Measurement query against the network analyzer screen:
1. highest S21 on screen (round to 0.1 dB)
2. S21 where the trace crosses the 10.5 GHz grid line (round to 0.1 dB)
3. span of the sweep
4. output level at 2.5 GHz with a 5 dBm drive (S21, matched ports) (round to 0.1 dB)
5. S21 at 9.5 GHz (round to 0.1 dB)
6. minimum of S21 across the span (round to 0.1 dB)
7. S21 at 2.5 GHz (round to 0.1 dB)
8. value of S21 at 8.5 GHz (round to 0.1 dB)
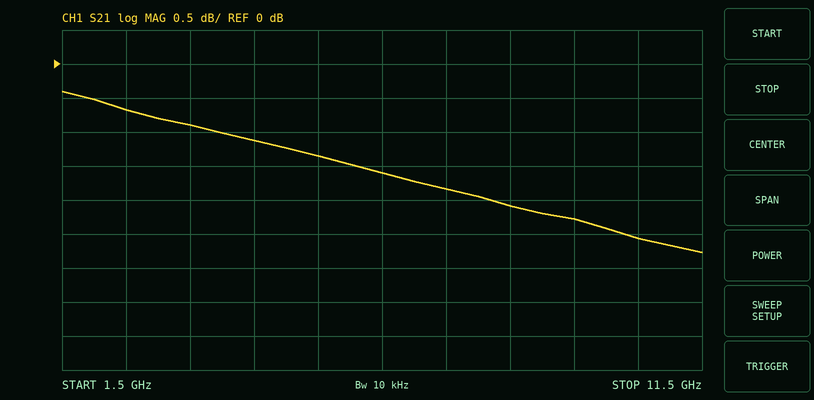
-0.4 dB
-2.6 dB
10 GHz
4.3 dBm
-2.3 dB
-2.8 dB
-0.7 dB
-2.1 dB
